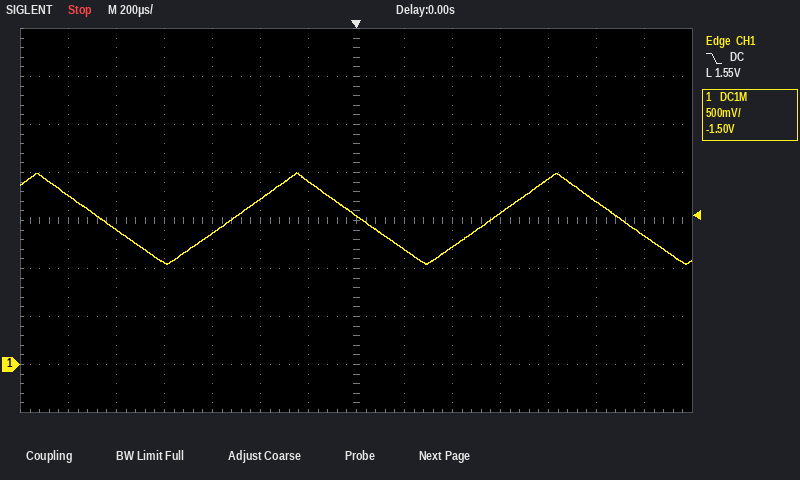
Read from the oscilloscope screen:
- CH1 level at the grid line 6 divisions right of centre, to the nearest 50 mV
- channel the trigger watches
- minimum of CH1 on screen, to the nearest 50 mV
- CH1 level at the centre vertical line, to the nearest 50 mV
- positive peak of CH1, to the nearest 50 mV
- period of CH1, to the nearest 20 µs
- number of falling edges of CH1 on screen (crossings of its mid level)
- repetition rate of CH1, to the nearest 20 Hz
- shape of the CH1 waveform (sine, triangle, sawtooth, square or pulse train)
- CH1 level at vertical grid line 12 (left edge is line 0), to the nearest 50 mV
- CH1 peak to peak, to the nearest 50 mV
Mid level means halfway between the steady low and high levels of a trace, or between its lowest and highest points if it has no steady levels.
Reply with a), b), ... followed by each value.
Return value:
a) 1.35 V
b) CH1
c) 1.05 V
d) 1.55 V
e) 2.00 V
f) 1.08 ms
g) 3
h) 920 Hz
i) triangle
j) 1.70 V
k) 950 mV
